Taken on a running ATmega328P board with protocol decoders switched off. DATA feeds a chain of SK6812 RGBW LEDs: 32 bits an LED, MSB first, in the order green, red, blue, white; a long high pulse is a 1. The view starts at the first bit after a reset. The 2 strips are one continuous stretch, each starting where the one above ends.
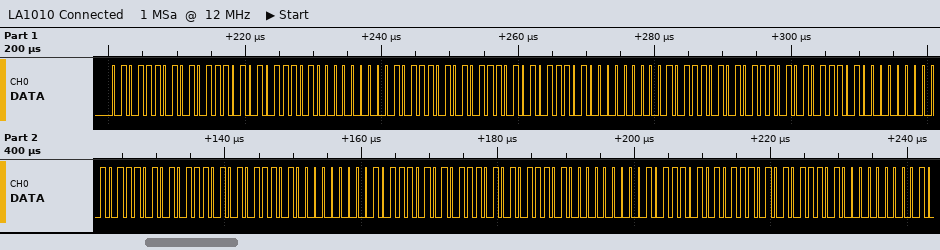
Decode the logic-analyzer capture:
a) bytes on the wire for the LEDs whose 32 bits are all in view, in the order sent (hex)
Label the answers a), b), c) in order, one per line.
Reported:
a) 5D 5D 5D 00 5D 5D 5D 00 5D 5D 5D 00 5D 5D 5D 00 5D 5D 5D 00 5D 5D 5D 00
